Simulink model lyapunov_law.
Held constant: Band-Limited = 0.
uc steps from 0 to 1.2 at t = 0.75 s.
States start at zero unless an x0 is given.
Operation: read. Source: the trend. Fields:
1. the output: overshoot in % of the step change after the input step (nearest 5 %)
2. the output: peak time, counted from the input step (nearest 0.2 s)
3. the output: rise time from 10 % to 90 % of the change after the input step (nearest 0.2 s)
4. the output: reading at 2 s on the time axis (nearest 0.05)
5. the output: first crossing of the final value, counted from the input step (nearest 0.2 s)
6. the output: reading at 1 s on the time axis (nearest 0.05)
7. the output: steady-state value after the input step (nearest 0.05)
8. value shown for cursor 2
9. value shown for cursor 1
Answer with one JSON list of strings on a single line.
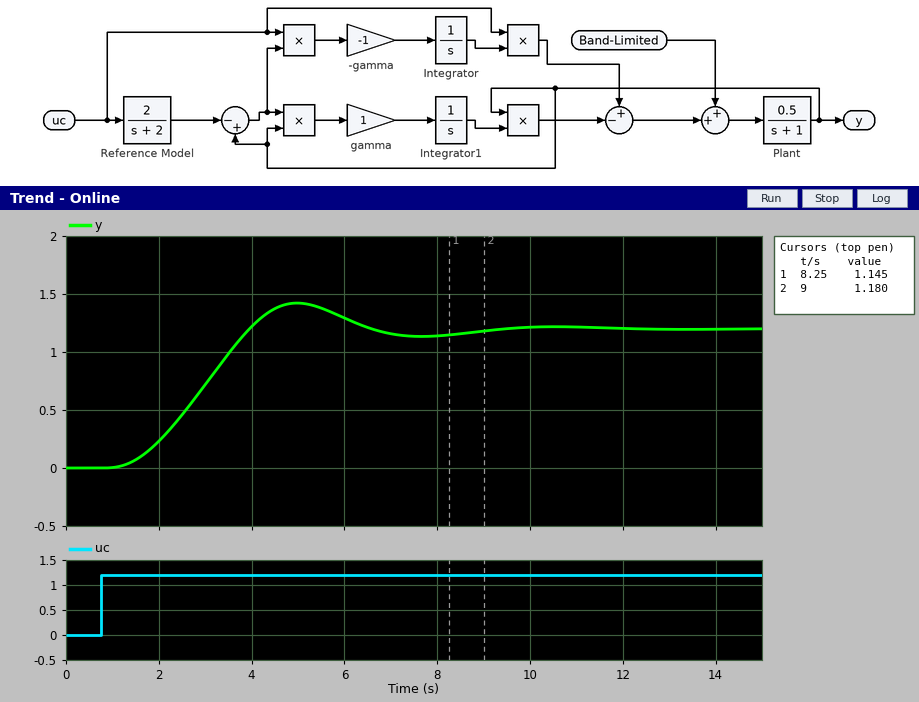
["20 %", "4.2 s", "2.0 s", "0.25", "3.2 s", "0.00", "1.20", "1.180", "1.145"]
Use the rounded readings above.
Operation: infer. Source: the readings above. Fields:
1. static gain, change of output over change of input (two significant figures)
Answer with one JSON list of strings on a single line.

["1.0"]
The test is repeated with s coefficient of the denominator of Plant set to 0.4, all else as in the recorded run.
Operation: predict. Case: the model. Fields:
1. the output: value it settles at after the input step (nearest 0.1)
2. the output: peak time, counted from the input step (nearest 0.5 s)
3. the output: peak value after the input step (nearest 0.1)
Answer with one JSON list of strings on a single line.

["1.2", "3.5 s", "1.3"]
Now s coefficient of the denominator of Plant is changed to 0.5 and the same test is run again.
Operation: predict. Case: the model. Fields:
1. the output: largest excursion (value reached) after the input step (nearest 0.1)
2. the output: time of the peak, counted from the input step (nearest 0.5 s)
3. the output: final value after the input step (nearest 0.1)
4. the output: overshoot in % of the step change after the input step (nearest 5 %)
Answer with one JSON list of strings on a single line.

["1.3", "3.5 s", "1.2", "10 %"]
